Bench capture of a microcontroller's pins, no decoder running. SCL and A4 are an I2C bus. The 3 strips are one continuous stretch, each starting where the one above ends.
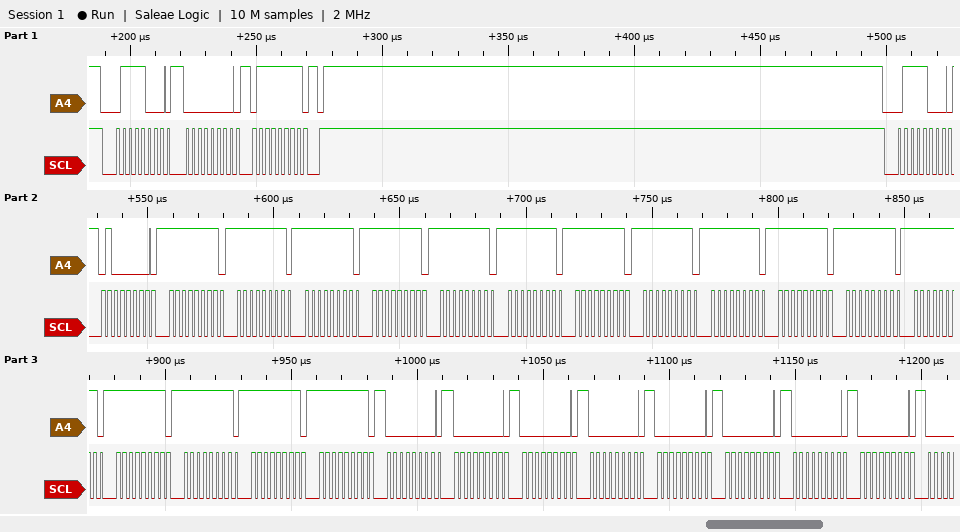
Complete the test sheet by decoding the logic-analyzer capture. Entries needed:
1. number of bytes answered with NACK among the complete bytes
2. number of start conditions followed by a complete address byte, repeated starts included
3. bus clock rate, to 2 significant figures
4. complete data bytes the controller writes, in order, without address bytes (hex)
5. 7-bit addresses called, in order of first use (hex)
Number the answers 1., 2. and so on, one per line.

1. 0
2. 2
3. 400 kHz
4. 00 7F 40 FF FF FF FF FF FF FF FF FF FF FF FF FF FF FF FF 00 00 00 00 00 00 00 00
5. 0x3C
